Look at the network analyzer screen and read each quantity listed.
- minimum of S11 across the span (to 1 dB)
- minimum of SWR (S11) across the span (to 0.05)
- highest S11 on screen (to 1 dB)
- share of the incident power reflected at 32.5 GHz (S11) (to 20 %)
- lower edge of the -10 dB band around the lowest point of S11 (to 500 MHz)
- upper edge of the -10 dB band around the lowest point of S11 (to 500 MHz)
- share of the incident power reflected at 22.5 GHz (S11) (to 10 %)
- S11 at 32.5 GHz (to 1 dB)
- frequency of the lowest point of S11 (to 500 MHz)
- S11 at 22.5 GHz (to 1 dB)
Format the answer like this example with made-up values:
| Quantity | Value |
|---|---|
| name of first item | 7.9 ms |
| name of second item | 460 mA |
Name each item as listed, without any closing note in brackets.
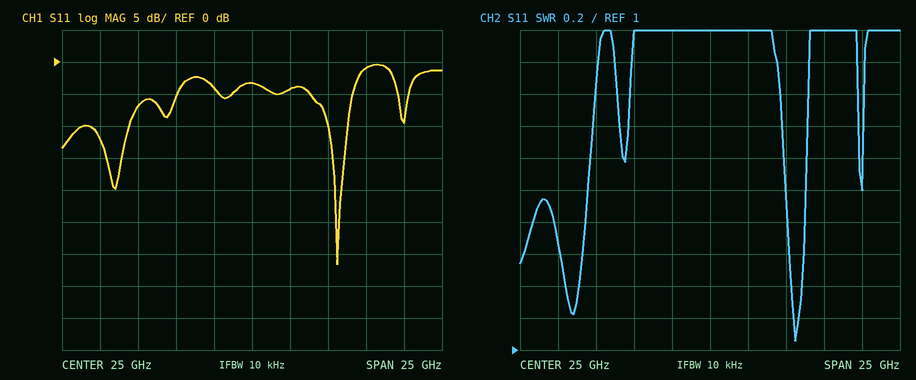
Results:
| Quantity | Value |
|---|---|
| minimum of S11 across the span | -32 dB |
| minimum of SWR (S11) across the span | 1.05 |
| highest S11 on screen | 0 dB |
| share of the incident power reflected at 32.5 GHz (S11) | 80 % |
| lower edge of the -10 dB band around the lowest point of S11 | 30.0 GHz |
| upper edge of the -10 dB band around the lowest point of S11 | 31.5 GHz |
| share of the incident power reflected at 22.5 GHz (S11) | 40 % |
| S11 at 32.5 GHz | -1 dB |
| frequency of the lowest point of S11 | 30.5 GHz |
| S11 at 22.5 GHz | -4 dB |
